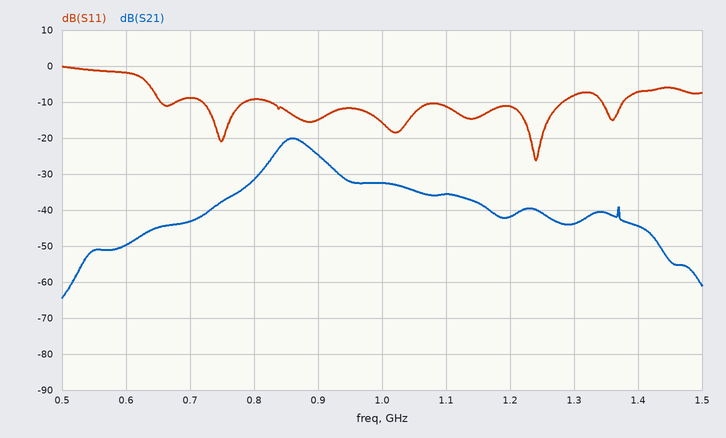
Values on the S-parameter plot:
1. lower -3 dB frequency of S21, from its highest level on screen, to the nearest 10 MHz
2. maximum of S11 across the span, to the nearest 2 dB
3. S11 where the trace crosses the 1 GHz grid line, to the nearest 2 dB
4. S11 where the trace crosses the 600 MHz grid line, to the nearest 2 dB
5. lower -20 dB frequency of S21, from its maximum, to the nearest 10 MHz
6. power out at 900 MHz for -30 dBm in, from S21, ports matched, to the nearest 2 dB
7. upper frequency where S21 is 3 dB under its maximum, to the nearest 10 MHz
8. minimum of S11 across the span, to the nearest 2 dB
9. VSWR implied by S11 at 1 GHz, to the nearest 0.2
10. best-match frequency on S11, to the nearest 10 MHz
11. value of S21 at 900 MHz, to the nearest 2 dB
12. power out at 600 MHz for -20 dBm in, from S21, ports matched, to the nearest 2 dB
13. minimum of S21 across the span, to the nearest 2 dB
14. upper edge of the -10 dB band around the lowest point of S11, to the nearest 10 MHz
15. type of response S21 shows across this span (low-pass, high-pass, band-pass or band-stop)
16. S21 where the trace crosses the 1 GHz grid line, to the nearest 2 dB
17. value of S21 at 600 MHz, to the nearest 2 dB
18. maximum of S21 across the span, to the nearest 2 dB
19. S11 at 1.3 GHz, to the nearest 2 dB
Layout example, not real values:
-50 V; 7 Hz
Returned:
840 MHz; 0 dB; -16 dB; -2 dB; 730 MHz; -54 dBm; 890 MHz; -26 dB; 1.4; 1.24 GHz; -24 dB; -70 dBm; -64 dB; 1.28 GHz; band-pass; -32 dB; -50 dB; -20 dB; -8 dB
